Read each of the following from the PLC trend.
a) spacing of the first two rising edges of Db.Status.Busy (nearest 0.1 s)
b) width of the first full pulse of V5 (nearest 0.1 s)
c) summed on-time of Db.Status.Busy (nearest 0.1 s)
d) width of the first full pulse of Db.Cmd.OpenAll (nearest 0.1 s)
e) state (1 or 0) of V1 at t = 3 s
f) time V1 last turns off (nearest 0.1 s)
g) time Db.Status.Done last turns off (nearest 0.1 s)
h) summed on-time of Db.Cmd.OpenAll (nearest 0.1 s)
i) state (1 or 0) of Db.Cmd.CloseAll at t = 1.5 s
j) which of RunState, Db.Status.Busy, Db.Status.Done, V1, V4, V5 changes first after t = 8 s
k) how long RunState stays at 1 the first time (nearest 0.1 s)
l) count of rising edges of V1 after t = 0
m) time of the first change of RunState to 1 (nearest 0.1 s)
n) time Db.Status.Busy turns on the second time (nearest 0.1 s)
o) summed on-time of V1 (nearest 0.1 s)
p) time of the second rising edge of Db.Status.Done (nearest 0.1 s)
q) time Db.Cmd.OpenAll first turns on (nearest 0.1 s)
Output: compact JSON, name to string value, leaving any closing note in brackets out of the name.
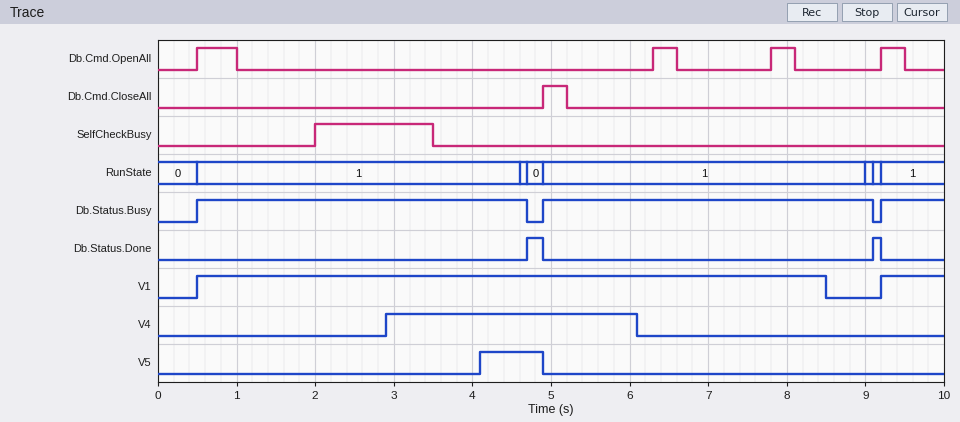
{"spacing of the first two rising edges of Db.Status.Busy": "4.4 s", "width of the first full pulse of V5": "0.8 s", "summed on-time of Db.Status.Busy": "9.2 s", "width of the first full pulse of Db.Cmd.OpenAll": "0.5 s", "state (1 or 0) of V1 at t = 3 s": "1", "time V1 last turns off": "8.5 s", "time Db.Status.Done last turns off": "9.2 s", "summed on-time of Db.Cmd.OpenAll": "1.4 s", "state (1 or 0) of Db.Cmd.CloseAll at t = 1.5 s": "0", "which of RunState, Db.Status.Busy, Db.Status.Done, V1, V4, V5 changes first after t = 8 s": "V1", "how long RunState stays at 1 the first time": "4.1 s", "count of rising edges of V1 after t = 0": "2", "time of the first change of RunState to 1": "0.5 s", "time Db.Status.Busy turns on the second time": "4.9 s", "summed on-time of V1": "8.8 s", "time of the second rising edge of Db.Status.Done": "9.1 s", "time Db.Cmd.OpenAll first turns on": "0.5 s"}
